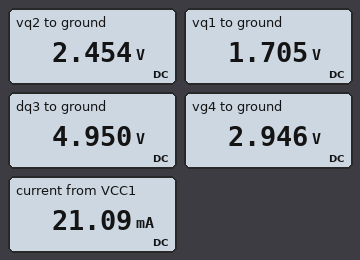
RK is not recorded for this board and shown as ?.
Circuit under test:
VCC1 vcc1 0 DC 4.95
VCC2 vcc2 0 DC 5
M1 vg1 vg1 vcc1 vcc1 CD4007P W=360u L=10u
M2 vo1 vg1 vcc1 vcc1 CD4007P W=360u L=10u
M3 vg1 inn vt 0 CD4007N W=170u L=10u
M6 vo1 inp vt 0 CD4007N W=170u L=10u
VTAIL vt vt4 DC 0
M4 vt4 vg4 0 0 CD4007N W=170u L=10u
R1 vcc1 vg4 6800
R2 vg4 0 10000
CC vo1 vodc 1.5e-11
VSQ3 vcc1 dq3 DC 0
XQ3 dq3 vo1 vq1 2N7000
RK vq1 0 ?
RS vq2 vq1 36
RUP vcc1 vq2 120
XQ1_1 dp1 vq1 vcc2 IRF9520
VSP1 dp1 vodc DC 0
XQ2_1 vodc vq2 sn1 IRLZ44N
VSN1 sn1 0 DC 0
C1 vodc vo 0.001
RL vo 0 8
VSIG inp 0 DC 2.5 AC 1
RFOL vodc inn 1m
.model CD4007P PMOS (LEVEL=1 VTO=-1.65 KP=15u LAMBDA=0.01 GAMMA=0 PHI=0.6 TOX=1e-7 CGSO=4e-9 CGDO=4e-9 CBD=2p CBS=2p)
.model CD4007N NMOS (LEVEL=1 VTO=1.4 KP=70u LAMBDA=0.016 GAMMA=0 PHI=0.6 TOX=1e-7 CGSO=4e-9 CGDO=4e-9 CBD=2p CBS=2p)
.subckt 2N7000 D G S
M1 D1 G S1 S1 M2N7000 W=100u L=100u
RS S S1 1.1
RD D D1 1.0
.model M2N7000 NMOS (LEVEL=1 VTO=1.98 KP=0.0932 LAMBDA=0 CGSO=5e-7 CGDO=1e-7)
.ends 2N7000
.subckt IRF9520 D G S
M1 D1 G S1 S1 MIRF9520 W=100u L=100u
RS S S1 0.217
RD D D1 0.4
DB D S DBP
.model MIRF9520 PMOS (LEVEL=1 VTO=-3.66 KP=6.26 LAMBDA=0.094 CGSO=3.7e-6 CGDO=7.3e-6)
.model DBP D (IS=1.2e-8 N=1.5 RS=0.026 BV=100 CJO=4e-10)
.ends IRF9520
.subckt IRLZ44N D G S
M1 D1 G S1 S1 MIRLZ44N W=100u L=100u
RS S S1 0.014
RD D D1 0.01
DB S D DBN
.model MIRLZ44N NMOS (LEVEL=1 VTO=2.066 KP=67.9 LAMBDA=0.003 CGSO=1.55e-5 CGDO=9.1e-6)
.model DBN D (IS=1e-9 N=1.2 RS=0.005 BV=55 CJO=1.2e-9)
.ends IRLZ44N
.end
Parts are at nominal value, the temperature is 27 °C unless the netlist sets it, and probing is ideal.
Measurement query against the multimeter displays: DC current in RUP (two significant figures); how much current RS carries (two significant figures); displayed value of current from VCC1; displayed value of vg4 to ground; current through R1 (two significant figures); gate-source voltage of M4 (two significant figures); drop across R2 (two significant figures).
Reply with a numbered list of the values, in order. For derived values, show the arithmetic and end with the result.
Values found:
1. (4.95 V - 2.454 V) / 120 Ω = 21 mA
2. (2.454 V - 1.705 V) / 36 Ω = 21 mA
3. 21.09 mA
4. 2.946 V
5. (4.95 V - 2.946 V) / 6.8 kΩ = 290 µA
6. 2.946 V = 2.9 V
7. 2.946 V = 2.9 V
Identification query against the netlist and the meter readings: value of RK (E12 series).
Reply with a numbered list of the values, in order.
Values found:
1. 82 Ω
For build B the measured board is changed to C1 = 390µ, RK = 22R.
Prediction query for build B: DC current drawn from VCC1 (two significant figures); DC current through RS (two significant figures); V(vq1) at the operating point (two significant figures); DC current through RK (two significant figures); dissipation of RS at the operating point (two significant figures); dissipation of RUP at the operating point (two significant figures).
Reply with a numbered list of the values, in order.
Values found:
1. 57 mA
2. 24 mA
3. 1.2 V
4. 56 mA
5. 20 mW
6. 68 mW
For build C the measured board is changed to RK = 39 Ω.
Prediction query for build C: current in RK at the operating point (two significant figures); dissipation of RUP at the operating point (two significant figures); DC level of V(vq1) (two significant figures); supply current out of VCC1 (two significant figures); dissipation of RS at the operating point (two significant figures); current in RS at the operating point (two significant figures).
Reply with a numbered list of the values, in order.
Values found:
1. 32 mA
2. 68 mW
3. 1.2 V
4. 33 mA
5. 20 mW
6. 24 mA
